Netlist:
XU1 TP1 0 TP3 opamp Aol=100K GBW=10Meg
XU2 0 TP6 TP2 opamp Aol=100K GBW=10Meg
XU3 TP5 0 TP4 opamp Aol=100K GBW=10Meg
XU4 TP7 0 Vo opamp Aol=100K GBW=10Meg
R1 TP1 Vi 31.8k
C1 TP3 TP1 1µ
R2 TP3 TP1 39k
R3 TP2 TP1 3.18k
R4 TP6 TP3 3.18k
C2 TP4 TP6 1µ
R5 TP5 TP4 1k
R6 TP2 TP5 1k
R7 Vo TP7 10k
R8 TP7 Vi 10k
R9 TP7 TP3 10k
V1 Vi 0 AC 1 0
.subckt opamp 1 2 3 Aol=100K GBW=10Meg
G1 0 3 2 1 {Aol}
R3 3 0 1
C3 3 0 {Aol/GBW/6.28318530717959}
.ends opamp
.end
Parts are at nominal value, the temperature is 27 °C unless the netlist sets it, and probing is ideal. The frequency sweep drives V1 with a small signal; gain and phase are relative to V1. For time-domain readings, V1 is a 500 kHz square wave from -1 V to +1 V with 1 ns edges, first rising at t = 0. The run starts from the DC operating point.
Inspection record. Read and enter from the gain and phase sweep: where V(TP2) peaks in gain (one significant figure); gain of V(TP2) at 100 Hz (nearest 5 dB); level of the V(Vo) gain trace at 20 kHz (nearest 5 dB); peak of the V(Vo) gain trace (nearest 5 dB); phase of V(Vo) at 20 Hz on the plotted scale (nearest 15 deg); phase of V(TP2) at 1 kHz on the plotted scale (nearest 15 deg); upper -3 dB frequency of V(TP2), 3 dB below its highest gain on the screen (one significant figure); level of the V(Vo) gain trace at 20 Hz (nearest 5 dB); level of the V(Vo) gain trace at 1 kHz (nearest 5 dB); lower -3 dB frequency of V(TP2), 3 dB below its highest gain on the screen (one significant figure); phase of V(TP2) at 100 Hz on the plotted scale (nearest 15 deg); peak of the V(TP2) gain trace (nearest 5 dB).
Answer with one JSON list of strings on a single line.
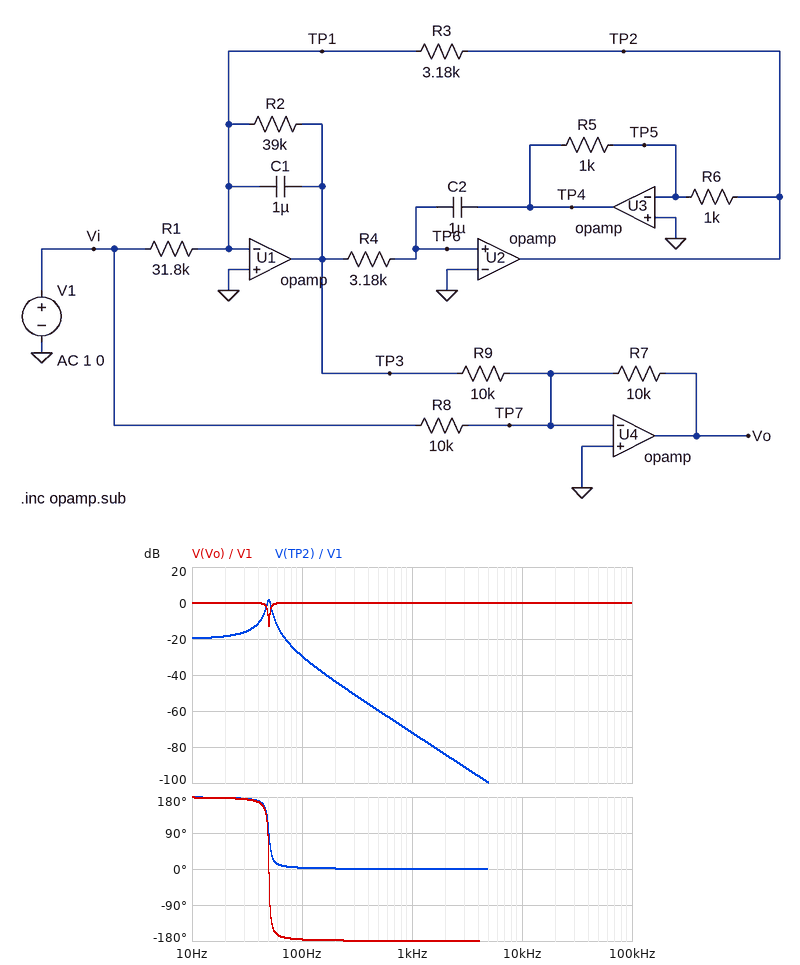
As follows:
["50 Hz", "-30 dB", "0 dB", "0 dB", "180 deg", "0 deg", "50 Hz", "0 dB", "0 dB", "50 Hz", "0 deg", "0 dB"]
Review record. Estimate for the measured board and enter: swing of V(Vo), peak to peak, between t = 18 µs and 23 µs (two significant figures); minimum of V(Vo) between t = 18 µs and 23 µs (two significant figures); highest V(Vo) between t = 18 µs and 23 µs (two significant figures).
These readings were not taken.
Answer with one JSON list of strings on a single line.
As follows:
["2.0 V", "-1.0 V", "1.0 V"]
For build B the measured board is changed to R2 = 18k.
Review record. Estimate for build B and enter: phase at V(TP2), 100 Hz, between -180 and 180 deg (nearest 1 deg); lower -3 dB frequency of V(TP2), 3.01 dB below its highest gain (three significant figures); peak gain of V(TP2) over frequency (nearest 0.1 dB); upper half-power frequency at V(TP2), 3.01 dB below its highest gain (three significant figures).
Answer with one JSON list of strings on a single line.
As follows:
["7 deg", "45.0 Hz", "-4.9 dB", "53.9 Hz"]
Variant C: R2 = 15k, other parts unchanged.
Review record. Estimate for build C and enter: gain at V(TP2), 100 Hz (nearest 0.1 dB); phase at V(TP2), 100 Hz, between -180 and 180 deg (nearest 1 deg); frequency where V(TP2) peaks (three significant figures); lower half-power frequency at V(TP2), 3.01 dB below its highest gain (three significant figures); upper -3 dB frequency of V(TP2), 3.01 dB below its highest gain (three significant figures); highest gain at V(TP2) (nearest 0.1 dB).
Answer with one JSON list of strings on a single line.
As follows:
["-29.6 dB", "8 deg", "49.5 Hz", "43.8 Hz", "54.6 Hz", "-6.5 dB"]
